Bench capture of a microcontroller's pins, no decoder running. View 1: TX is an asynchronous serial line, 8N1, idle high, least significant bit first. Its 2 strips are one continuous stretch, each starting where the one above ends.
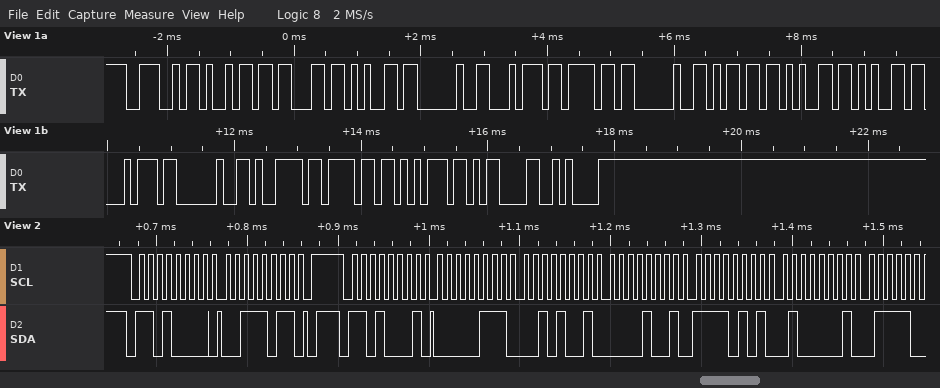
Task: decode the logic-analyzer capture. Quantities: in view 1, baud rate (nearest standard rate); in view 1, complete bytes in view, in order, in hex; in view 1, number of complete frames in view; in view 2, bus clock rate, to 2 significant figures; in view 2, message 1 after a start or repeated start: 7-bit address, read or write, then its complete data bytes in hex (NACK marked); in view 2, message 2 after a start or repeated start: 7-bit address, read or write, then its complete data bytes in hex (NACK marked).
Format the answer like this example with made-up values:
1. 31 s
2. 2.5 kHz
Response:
1. 9600 baud
2. 4E 69 63 65 20 74 6F 20 6D 65 65 74 20 79 6F 75 0D 0A
3. 18
4. 100 kHz
5. 0x68 write: 3B
6. 0x68 read: 07 29 09 F5 41
